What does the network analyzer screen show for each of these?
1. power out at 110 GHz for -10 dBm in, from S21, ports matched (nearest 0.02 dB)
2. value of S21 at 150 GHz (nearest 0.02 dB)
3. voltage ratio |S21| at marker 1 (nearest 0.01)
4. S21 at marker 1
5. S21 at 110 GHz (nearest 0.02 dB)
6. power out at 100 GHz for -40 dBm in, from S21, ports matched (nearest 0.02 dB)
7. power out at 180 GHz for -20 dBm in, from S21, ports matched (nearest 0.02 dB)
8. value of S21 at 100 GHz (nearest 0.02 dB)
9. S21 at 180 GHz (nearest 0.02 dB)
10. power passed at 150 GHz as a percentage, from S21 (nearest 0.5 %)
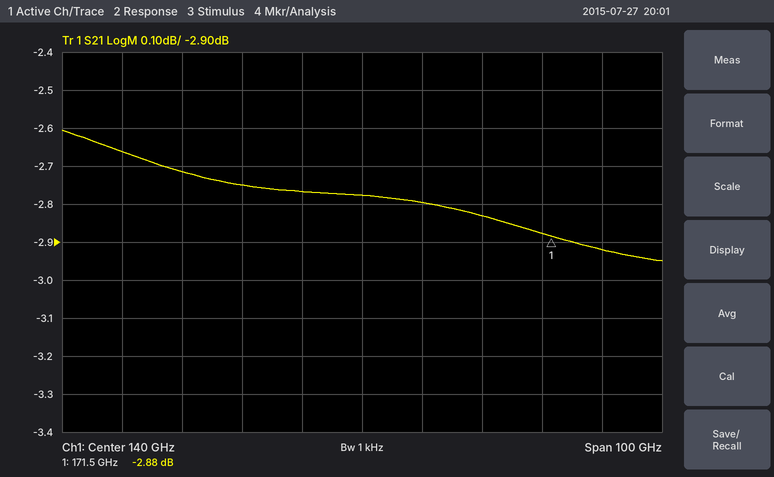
-12.72 dBm
-2.80 dB
0.72
-2.88 dB
-2.72 dB
-42.66 dBm
-22.92 dBm
-2.66 dB
-2.92 dB
52.5 %
